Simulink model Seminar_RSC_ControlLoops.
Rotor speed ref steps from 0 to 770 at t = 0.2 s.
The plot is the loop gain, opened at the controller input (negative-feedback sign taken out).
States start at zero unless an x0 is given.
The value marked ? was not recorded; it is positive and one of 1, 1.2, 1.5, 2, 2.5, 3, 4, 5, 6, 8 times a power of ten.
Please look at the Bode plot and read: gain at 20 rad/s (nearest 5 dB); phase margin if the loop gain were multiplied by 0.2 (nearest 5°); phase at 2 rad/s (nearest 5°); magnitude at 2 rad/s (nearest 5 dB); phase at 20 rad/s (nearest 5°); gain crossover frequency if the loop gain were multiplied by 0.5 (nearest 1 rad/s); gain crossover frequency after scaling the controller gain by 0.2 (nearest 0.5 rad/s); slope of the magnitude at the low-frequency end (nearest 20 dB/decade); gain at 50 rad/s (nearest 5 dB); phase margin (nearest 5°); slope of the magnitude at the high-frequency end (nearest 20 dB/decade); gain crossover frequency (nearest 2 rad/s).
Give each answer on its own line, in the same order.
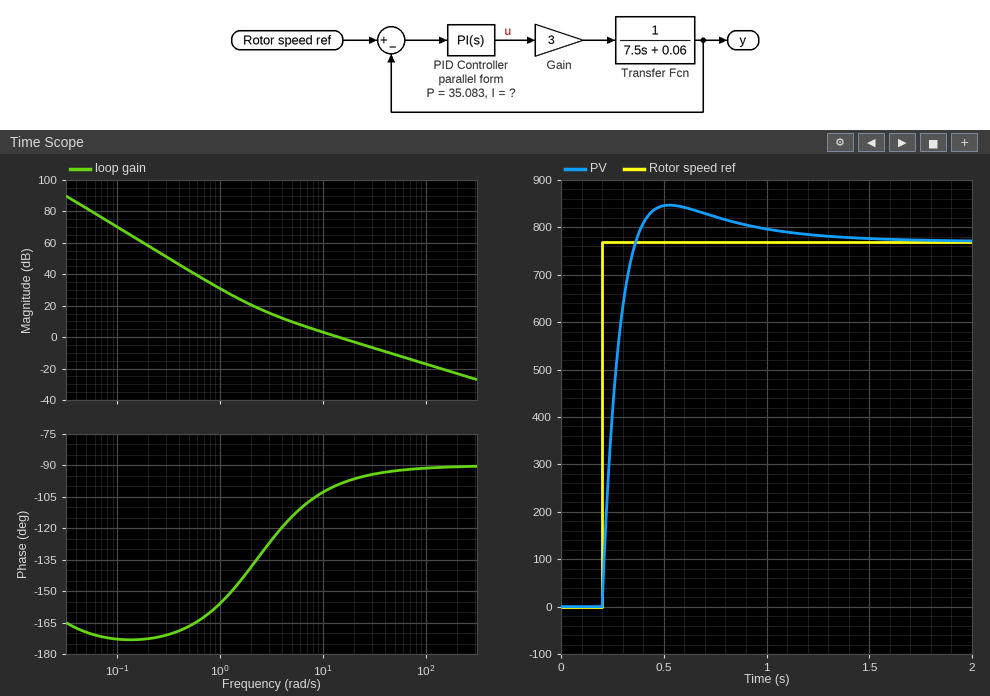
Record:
-5 dB
55°
-140°
20 dB
-95°
7 rad/s
3.5 rad/s
-40 dB/decade
-10 dB
80°
-20 dB/decade
14 rad/s
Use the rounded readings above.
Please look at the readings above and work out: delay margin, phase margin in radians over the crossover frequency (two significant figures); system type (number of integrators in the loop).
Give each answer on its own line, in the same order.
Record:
0.100 s
2
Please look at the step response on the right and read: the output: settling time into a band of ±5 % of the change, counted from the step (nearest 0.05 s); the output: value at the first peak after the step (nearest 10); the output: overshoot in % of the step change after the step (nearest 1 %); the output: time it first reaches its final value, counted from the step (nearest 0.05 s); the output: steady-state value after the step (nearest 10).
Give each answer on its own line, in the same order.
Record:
0.65 s
850
10 %
0.15 s
770
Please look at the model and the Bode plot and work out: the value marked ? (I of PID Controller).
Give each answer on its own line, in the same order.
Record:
80
